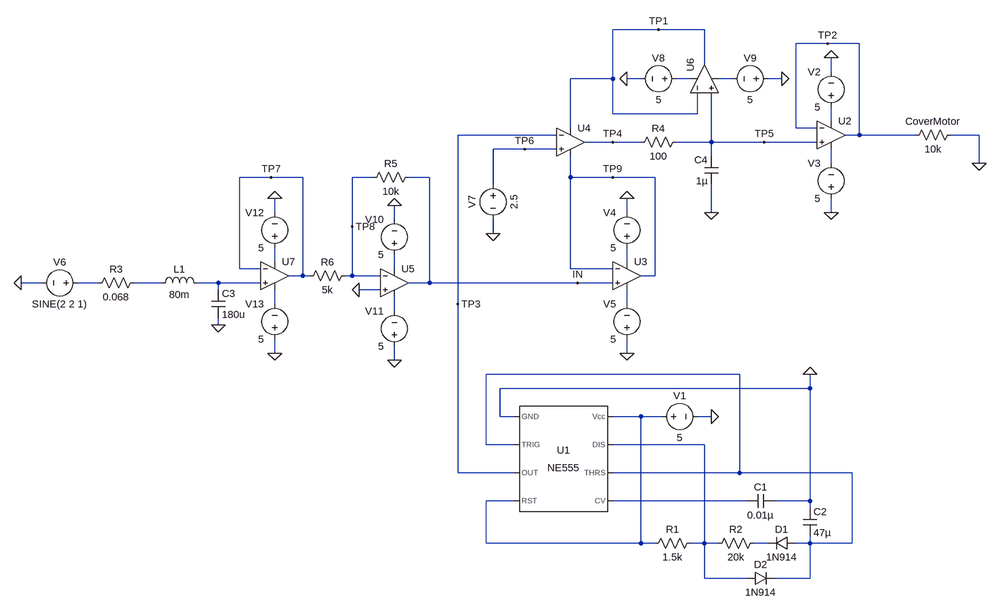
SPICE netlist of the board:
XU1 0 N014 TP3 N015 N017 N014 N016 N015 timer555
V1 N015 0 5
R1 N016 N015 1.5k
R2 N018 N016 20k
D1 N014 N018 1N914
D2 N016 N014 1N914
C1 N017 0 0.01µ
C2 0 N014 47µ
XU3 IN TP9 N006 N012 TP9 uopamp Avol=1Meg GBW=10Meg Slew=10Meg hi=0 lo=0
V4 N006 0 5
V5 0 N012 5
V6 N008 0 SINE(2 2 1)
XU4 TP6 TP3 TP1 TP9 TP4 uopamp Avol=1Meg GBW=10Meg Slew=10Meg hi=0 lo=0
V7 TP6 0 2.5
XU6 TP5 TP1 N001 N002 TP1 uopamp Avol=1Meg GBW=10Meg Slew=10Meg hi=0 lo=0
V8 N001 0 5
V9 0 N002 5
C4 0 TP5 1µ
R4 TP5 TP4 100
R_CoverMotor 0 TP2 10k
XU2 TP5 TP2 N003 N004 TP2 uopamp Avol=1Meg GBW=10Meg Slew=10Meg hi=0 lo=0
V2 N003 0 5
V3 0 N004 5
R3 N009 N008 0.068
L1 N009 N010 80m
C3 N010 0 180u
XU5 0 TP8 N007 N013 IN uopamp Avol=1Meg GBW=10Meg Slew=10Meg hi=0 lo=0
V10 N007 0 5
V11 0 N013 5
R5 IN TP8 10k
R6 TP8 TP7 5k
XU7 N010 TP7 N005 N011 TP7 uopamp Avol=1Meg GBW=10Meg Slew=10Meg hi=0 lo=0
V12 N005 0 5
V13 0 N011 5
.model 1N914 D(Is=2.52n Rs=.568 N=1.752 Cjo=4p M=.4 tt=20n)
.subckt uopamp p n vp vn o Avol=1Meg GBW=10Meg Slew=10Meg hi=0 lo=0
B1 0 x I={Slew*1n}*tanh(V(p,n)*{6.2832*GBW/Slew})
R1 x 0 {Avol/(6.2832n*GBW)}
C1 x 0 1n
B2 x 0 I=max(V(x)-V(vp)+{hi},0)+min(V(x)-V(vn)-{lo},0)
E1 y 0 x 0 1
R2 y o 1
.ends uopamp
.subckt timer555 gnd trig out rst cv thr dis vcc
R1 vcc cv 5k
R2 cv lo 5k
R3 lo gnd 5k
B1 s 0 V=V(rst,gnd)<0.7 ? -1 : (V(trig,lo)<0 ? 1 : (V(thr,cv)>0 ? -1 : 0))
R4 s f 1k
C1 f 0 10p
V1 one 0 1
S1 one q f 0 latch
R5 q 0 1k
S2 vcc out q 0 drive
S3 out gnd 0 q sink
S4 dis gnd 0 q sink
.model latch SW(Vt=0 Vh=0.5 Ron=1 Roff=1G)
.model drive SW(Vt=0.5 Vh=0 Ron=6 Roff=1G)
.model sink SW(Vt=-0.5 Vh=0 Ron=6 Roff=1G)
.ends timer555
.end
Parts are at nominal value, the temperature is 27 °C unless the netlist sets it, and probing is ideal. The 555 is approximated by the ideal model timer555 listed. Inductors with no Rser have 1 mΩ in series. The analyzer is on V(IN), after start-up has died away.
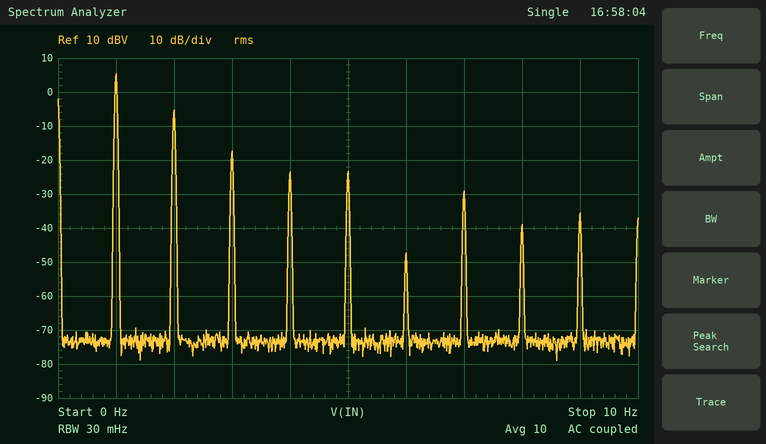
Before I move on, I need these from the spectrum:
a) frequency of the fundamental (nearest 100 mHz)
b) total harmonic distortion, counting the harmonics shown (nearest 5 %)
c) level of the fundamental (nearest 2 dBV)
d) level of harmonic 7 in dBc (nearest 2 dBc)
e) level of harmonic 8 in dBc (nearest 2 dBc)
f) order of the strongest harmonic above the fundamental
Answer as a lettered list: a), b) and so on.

a) 1.0 Hz
b) 30 %
c) 6 dBV
d) -34 dBc
e) -44 dBc
f) 2
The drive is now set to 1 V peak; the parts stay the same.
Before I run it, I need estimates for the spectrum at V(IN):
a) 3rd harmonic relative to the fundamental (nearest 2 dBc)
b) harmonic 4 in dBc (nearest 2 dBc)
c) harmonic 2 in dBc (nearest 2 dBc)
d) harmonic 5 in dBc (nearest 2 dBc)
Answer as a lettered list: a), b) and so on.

a) -22 dBc
b) -36 dBc
c) -16 dBc
d) -36 dBc
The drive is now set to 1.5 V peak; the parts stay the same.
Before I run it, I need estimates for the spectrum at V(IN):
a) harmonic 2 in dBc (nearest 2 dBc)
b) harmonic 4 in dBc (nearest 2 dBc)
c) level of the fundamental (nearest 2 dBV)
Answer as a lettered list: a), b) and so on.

a) -12 dBc
b) -36 dBc
c) 4 dBV
